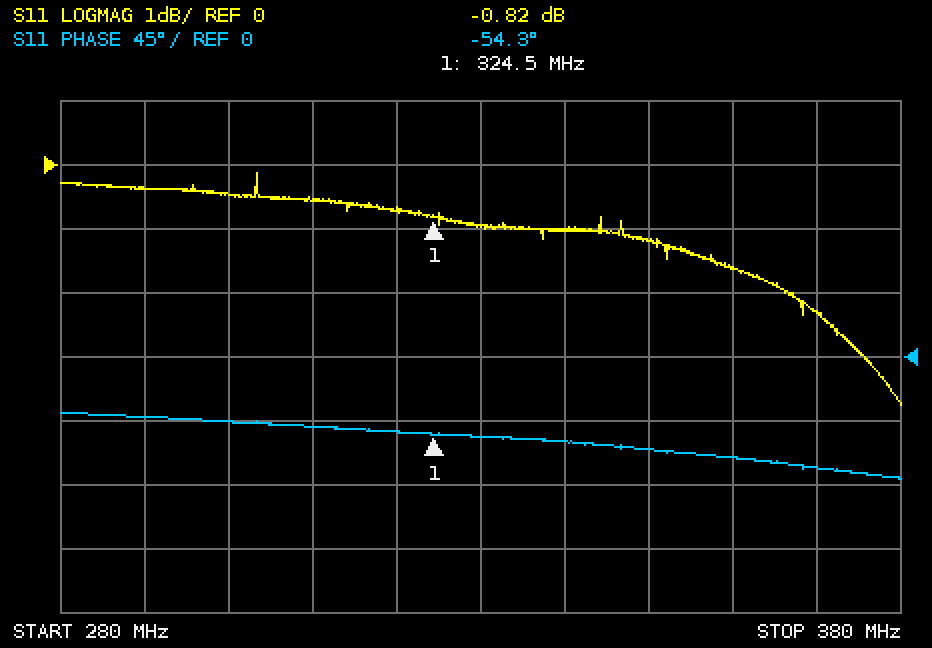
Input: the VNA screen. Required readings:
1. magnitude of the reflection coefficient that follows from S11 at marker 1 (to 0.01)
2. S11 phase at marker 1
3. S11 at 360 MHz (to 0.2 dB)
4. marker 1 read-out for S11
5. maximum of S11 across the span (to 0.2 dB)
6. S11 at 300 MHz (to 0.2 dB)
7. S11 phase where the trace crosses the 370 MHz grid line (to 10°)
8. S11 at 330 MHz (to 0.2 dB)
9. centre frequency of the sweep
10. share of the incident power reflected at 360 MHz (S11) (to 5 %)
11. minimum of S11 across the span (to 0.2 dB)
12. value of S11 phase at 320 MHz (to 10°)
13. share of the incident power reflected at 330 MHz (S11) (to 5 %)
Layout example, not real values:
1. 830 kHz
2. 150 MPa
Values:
1. 0.91
2. -54.3°
3. -1.6 dB
4. -0.82 dB
5. -0.2 dB
6. -0.4 dB
7. -80°
8. -1.0 dB
9. 330 MHz
10. 70 %
11. -3.8 dB
12. -50°
13. 80 %
